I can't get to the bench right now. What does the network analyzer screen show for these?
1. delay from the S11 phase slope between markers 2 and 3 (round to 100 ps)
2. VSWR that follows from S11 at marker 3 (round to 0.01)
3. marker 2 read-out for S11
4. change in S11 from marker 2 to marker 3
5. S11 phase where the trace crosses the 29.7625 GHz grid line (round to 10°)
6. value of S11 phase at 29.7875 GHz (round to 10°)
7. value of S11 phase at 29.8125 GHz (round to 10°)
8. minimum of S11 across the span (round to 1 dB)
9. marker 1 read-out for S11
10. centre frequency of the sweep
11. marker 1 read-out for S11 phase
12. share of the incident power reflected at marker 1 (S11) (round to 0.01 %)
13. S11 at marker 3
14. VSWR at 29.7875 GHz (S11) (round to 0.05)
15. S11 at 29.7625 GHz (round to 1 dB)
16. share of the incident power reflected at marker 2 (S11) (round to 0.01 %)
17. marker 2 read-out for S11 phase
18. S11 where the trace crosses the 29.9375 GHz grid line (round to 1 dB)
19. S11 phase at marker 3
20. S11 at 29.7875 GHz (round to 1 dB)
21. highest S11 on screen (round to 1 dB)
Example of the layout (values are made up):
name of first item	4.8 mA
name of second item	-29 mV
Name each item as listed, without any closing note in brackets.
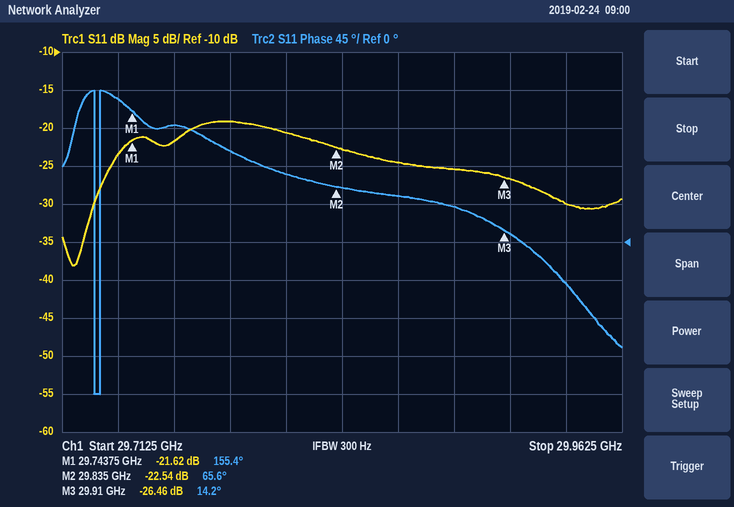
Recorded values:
delay from the S11 phase slope between markers 2 and 3	1.9 ns
VSWR that follows from S11 at marker 3	1.10
marker 2 read-out for S11	-22.54 dB
change in S11 from marker 2 to marker 3	-3.92 dB
S11 phase where the trace crosses the 29.7625 GHz grid line	140°
value of S11 phase at 29.7875 GHz	110°
value of S11 phase at 29.8125 GHz	80°
minimum of S11 across the span	-38 dB
marker 1 read-out for S11	-21.62 dB
centre frequency of the sweep	29.8375 GHz
marker 1 read-out for S11 phase	155.4°
share of the incident power reflected at marker 1 (S11)	0.69 %
S11 at marker 3	-26.46 dB
VSWR at 29.7875 GHz (S11)	1.25
S11 at 29.7625 GHz	-22 dB
share of the incident power reflected at marker 2 (S11)	0.56 %
marker 2 read-out for S11 phase	65.6°
S11 where the trace crosses the 29.9375 GHz grid line	-30 dB
S11 phase at marker 3	14.2°
S11 at 29.7875 GHz	-19 dB
highest S11 on screen	-19 dB
